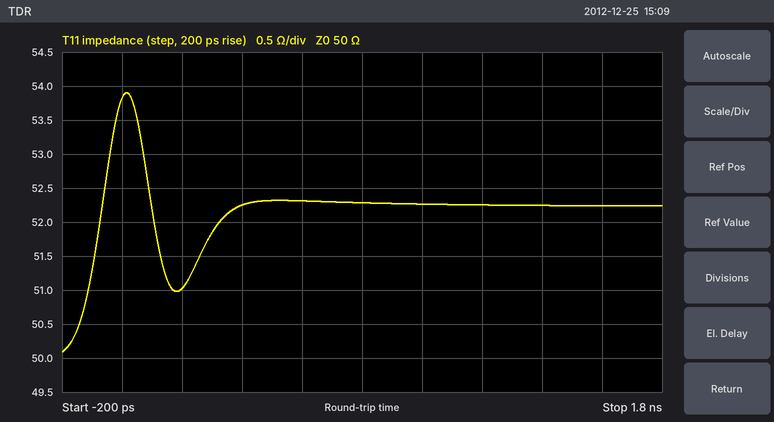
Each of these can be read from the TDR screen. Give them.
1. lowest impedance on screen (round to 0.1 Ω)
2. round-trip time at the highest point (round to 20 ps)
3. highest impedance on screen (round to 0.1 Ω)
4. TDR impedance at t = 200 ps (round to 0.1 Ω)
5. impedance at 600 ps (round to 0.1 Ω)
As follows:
50.1 Ω
20 ps
53.9 Ω
51.0 Ω
52.3 Ω
